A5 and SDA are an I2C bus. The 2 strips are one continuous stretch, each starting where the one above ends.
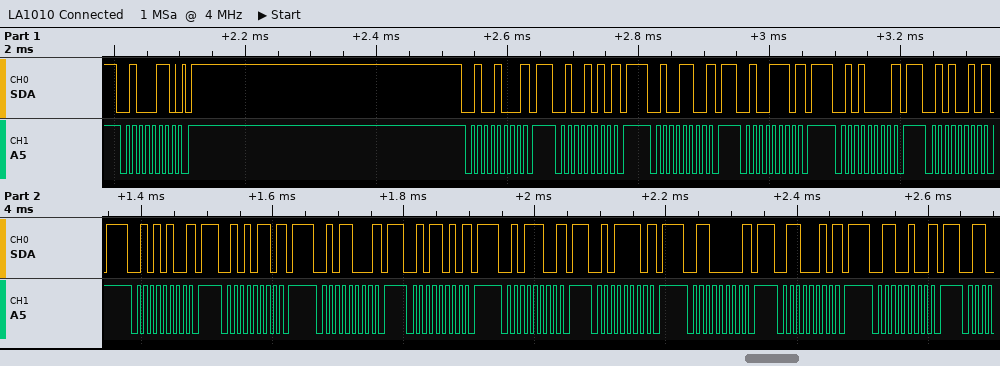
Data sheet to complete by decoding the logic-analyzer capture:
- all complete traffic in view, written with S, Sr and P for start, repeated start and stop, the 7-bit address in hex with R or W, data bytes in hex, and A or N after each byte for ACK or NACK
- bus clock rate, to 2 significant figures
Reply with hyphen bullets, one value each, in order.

- S 23W A P S 24W N P S 25W N P S 26W N P S 27W N P S 28W N P S 29W N P S 2AW N P S 2BW N P S 2CW N P S 2DW N P S 2EW N P S 2FW N P S 30W N P S 31W N P S 32W N P
- 100 kHz
